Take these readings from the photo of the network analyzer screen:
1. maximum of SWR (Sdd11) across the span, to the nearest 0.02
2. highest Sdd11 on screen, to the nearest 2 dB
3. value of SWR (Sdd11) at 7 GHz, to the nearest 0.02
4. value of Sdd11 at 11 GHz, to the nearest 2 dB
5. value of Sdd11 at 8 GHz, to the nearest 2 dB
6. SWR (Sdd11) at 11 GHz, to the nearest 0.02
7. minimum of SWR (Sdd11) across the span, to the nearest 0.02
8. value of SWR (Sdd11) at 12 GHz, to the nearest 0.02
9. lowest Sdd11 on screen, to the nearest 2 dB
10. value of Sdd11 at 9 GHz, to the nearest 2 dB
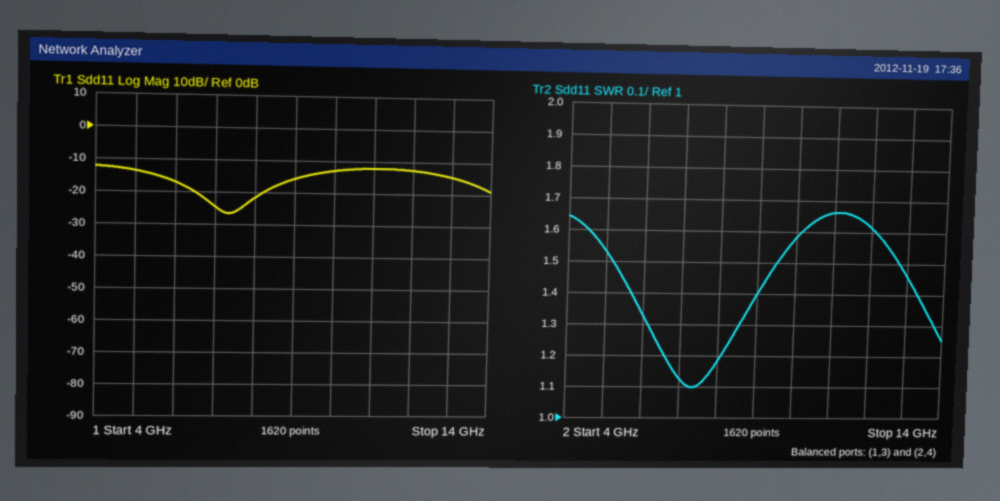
1.66
-12 dB
1.12
-12 dB
-22 dB
1.66
1.10
1.62
-26 dB
-16 dB
